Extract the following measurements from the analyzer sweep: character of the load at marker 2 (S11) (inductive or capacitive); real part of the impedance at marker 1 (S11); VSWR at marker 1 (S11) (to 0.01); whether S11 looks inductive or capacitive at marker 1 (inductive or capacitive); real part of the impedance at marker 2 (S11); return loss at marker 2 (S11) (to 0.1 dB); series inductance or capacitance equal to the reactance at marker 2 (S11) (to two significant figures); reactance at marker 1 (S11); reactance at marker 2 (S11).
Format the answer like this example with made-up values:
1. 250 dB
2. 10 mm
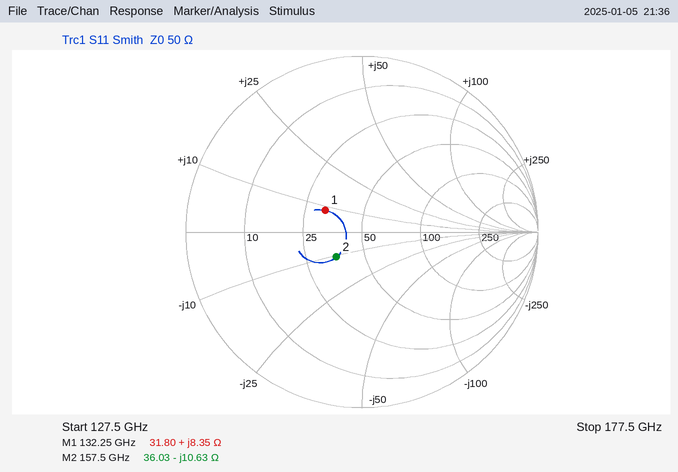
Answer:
1. capacitive
2. 31.80 Ω
3. 1.64
4. inductive
5. 36.03 Ω
6. 13.9 dB
7. 95 fF
8. +8.35 Ω
9. -10.63 Ω
